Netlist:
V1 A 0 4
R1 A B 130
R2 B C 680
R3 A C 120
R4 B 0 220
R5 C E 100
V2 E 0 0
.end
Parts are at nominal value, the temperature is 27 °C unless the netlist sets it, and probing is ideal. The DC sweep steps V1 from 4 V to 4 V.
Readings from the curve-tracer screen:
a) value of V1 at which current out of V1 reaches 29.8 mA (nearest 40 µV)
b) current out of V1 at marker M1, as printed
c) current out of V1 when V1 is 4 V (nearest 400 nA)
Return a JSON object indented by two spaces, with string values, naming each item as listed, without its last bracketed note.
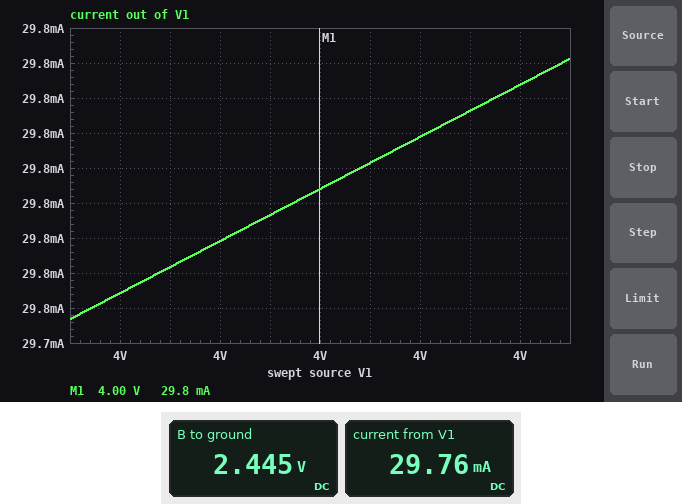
{
  "value of V1 at which current out of V1 reaches 29.8 mA": "4.00044 V",
  "current out of V1 at marker M1, as printed": "29.8 mA",
  "current out of V1 when V1 is 4 V": "29.7544 mA"
}
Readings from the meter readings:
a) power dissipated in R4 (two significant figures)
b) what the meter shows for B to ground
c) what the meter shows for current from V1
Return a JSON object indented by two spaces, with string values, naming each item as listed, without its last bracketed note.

{
  "power dissipated in R4": "27 mW",
  "what the meter shows for B to ground": "2.445 V",
  "what the meter shows for current from V1": "29.76 mA"
}
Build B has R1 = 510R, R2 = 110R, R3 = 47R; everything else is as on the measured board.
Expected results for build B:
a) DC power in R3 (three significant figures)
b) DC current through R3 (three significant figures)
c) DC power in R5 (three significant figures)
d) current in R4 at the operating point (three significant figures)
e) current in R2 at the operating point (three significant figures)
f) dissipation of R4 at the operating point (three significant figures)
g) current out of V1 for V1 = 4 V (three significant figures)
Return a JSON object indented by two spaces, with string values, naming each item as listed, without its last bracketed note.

{
  "DC power in R3": "44.3 mW",
  "DC current through R3": "30.7 mA",
  "DC power in R5": "65.4 mW",
  "current in R4 at the operating point": "9.06 mA",
  "current in R2 at the operating point": "5.13 mA",
  "dissipation of R4 at the operating point": "18.1 mW",
  "current out of V1 for V1 = 4 V": "34.6 mA"
}
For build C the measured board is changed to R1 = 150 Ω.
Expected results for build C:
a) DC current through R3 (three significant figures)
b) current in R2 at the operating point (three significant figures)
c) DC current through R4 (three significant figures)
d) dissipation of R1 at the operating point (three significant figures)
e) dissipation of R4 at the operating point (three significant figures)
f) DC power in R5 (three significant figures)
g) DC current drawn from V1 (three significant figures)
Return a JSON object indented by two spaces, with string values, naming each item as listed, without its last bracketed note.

{
  "DC current through R3": "17.9 mA",
  "current in R2 at the operating point": "680 µA",
  "DC current through R4": "10.5 mA",
  "dissipation of R1 at the operating point": "18.9 mW",
  "dissipation of R4 at the operating point": "24.4 mW",
  "DC power in R5": "34.4 mW",
  "DC current drawn from V1": "29.1 mA"
}
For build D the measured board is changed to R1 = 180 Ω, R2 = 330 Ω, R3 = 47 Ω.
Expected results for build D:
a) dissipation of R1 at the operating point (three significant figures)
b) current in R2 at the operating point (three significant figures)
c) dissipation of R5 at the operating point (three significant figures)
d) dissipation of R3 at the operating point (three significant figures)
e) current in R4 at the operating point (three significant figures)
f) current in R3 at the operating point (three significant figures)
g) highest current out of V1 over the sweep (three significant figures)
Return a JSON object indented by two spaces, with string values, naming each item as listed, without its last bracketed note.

{
  "dissipation of R1 at the operating point": "15.8 mW",
  "current in R2 at the operating point": "1.13 mA",
  "dissipation of R5 at the operating point": "72.1 mW",
  "dissipation of R3 at the operating point": "36.8 mW",
  "current in R4 at the operating point": "10.5 mA",
  "current in R3 at the operating point": "28.0 mA",
  "highest current out of V1 over the sweep": "37.4 mA"
}
